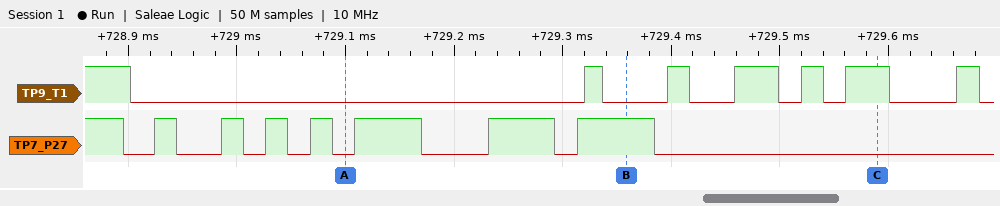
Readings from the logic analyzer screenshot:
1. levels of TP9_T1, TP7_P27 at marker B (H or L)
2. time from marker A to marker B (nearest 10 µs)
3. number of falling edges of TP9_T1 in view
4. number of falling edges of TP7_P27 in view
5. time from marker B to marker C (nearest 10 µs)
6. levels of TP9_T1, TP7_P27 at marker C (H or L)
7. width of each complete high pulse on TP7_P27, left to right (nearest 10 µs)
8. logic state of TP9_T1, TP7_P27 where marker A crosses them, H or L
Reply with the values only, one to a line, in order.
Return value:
TP9_T1=L, TP7_P27=H
260 µs
7
8
230 µs
TP9_T1=H, TP7_P27=L
20 µs, 20 µs, 20 µs, 20 µs, 60 µs, 60 µs, 70 µs
TP9_T1=L, TP7_P27=L
